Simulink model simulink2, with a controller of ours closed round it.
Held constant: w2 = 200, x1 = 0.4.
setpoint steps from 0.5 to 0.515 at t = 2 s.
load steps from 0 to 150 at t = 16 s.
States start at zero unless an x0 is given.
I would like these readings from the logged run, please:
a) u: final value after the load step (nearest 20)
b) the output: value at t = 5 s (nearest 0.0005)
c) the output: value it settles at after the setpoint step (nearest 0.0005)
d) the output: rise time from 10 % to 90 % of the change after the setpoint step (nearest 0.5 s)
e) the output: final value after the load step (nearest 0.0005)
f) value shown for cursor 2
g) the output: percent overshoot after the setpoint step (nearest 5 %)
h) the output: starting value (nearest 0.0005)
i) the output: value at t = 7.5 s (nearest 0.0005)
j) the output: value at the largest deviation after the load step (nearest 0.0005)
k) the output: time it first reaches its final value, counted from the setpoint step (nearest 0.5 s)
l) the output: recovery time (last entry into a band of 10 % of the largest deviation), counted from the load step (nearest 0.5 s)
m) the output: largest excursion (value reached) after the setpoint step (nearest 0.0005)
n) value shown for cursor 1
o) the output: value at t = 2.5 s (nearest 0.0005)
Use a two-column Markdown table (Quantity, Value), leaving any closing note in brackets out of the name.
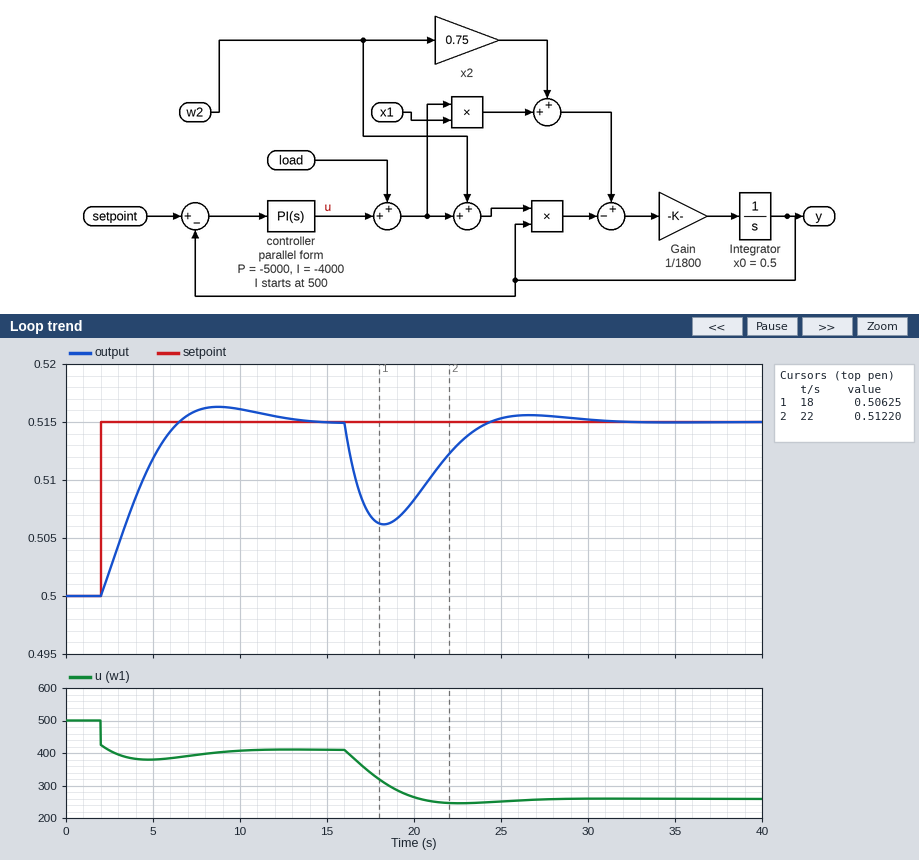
| Quantity | Value |
|---|---|
| u: final value after the load step | 260 |
| the output: value at t = 5 s | 0.5120 |
| the output: value it settles at after the setpoint step | 0.5150 |
| the output: rise time from 10 % to 90 % of the change after the setpoint step | 3.5 s |
| the output: final value after the load step | 0.5150 |
| value shown for cursor 2 | 0.51220 |
| the output: percent overshoot after the setpoint step | 10 % |
| the output: starting value | 0.5000 |
| the output: value at t = 7.5 s | 0.5160 |
| the output: value at the largest deviation after the load step | 0.5060 |
| the output: time it first reaches its final value, counted from the setpoint step | 4.5 s |
| the output: recovery time (last entry into a band of 10 % of the largest deviation), counted from the load step | 7.5 s |
| the output: largest excursion (value reached) after the setpoint step | 0.5165 |
| value shown for cursor 1 | 0.50625 |
| the output: value at t = 2.5 s | 0.5020 |
